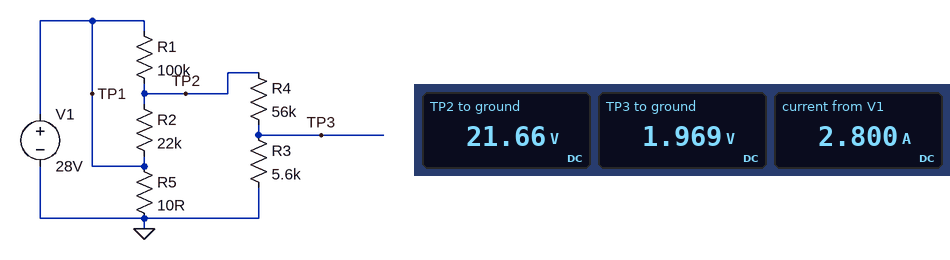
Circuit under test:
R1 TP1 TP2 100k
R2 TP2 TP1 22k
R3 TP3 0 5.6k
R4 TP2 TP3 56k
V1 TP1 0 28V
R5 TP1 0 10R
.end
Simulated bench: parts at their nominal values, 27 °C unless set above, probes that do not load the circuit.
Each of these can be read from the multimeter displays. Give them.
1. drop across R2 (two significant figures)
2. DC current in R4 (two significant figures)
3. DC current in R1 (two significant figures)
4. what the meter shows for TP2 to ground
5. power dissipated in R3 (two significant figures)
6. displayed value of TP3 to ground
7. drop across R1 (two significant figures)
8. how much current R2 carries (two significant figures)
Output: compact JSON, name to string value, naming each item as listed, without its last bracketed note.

{"drop across R2": "6.3 V", "DC current in R4": "350 µA", "DC current in R1": "63 µA", "what the meter shows for TP2 to ground": "21.66 V", "power dissipated in R3": "690 µW", "displayed value of TP3 to ground": "1.969 V", "drop across R1": "6.3 V", "how much current R2 carries": "290 µA"}
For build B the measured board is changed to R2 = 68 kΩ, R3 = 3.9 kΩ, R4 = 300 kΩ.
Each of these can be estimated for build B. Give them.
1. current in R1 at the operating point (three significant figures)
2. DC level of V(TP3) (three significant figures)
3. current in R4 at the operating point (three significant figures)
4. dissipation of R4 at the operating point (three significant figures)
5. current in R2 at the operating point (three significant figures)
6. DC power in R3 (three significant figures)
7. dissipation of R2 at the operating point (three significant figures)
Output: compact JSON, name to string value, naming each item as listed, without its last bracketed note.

{"current in R1 at the operating point": "32.9 µA", "DC level of V(TP3)": "317 mV", "current in R4 at the operating point": "81.3 µA", "dissipation of R4 at the operating point": "1.98 mW", "current in R2 at the operating point": "48.4 µA", "DC power in R3": "25.8 µW", "dissipation of R2 at the operating point": "159 µW"}
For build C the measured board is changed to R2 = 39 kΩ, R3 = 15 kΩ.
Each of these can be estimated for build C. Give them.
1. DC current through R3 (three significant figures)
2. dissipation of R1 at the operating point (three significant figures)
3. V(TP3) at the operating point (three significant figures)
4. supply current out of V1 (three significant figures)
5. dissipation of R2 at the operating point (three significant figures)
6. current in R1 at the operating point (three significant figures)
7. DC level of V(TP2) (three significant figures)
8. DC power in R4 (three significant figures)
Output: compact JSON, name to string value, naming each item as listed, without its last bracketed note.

{"DC current through R3": "283 µA", "dissipation of R1 at the operating point": "629 µW", "V(TP3) at the operating point": "4.24 V", "supply current out of V1": "2.80 A", "dissipation of R2 at the operating point": "1.61 mW", "current in R1 at the operating point": "79.3 µA", "DC level of V(TP2)": "20.1 V", "DC power in R4": "4.47 mW"}
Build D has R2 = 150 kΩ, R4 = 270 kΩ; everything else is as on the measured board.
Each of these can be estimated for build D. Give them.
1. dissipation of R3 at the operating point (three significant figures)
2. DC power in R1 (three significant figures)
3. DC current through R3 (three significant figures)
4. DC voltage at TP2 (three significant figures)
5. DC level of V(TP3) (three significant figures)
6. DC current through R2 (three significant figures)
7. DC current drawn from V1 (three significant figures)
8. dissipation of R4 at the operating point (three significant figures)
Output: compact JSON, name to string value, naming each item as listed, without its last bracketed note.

{"dissipation of R3 at the operating point": "39.0 µW", "DC power in R1": "251 µW", "DC current through R3": "83.4 µA", "DC voltage at TP2": "23.0 V", "DC level of V(TP3)": "467 mV", "DC current through R2": "33.4 µA", "DC current drawn from V1": "2.80 A", "dissipation of R4 at the operating point": "1.88 mW"}
